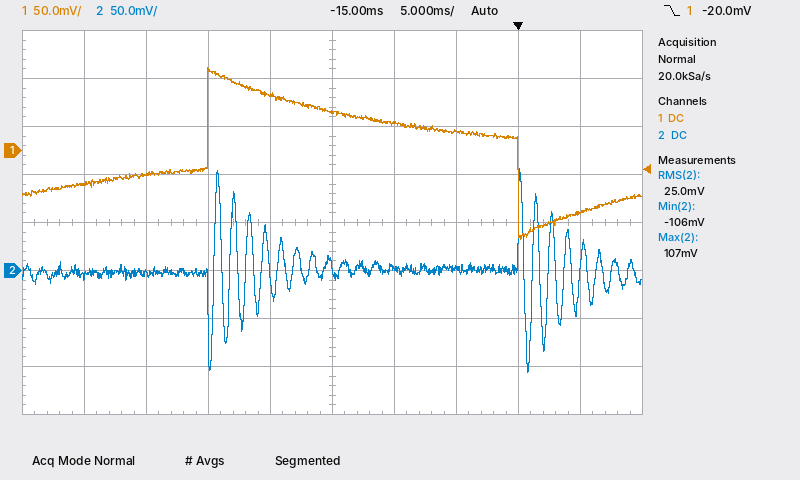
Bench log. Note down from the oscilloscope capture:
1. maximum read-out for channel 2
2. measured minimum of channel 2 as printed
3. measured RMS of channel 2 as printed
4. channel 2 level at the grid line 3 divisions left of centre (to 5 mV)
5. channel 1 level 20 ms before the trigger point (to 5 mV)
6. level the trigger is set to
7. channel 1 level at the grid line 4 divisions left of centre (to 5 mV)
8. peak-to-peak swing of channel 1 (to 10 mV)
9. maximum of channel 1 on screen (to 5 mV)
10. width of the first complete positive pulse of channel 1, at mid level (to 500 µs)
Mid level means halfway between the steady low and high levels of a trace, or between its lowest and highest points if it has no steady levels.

107 mV
-106 mV
25.0 mV
-5 mV
60 mV
-20.0 mV
-35 mV
180 mV
85 mV
25.0 ms
